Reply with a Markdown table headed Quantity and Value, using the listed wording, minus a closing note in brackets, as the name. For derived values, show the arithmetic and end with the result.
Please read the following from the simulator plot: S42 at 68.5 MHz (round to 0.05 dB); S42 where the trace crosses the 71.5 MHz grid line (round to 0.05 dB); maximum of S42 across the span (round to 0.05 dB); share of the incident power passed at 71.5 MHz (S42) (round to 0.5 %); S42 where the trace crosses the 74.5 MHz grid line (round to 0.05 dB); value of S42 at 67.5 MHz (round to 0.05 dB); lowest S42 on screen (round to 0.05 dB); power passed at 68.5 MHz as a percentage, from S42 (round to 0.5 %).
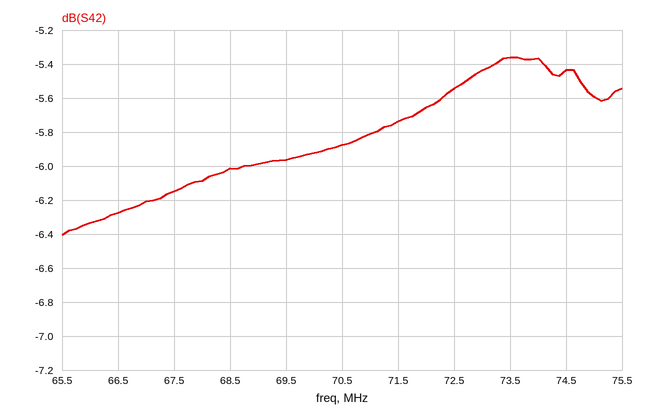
| Quantity | Value |
|---|---|
| S42 at 68.5 MHz | -6.00 dB |
| S42 where the trace crosses the 71.5 MHz grid line | -5.75 dB |
| maximum of S42 across the span | -5.35 dB |
| share of the incident power passed at 71.5 MHz (S42) | 10^(-5.75/10) ≈ 26.6 %, so 26.5 % to the nearest 0.5 % |
| S42 where the trace crosses the 74.5 MHz grid line | -5.45 dB |
| value of S42 at 67.5 MHz | -6.15 dB |
| lowest S42 on screen | -6.40 dB |
| power passed at 68.5 MHz as a percentage, from S42 | 10^(-6/10) ≈ 25.1 %, so 25.0 % to the nearest 0.5 % |
